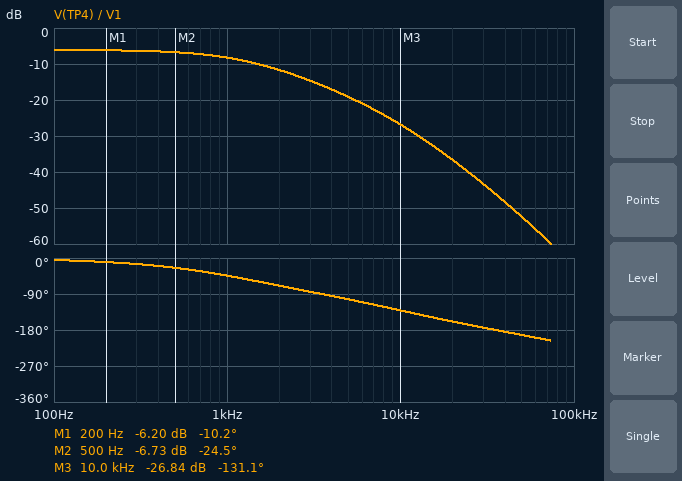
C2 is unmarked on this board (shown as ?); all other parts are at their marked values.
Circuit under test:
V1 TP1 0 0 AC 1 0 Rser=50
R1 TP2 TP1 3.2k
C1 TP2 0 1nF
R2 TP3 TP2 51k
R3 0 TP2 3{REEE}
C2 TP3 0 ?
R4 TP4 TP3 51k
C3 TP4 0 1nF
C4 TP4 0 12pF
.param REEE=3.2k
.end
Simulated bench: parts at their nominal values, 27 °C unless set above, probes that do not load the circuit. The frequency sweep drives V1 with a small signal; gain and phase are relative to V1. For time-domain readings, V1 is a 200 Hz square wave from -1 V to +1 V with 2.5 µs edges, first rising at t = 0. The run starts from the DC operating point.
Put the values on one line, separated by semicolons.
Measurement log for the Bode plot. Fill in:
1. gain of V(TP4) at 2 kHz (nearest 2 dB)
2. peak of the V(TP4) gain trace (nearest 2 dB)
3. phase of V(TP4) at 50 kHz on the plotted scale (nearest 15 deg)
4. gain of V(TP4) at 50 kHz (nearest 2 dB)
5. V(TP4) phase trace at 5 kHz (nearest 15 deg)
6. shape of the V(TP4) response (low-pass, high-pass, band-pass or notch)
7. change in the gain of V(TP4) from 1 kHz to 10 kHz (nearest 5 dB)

-12 dB; -6 dB; -195 deg; -52 dB; -105 deg; low-pass; -20 dB
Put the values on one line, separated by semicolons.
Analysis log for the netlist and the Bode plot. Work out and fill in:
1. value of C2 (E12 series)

680 pF
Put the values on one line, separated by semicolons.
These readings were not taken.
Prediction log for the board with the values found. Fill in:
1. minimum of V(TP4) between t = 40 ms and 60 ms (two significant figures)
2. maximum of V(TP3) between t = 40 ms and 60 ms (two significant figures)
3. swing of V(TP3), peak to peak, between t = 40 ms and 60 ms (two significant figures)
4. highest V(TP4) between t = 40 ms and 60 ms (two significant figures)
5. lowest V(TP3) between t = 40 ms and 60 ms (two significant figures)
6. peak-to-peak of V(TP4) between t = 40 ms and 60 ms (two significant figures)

-500 mV; 500 mV; 990 mV; 500 mV; -500 mV; 990 mV
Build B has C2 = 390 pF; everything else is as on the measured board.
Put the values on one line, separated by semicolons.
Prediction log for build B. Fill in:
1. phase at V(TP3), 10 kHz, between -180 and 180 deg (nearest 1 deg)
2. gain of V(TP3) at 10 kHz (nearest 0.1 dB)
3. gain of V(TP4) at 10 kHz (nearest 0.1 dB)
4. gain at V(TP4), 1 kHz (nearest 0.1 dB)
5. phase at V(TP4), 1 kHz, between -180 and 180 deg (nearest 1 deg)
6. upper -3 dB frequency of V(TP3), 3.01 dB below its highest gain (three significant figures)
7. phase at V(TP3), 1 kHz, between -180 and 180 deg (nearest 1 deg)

-45 deg; -14.1 dB; -24.7 dB; -8.0 dB; -40 deg; 1.73 kHz; -22 deg
